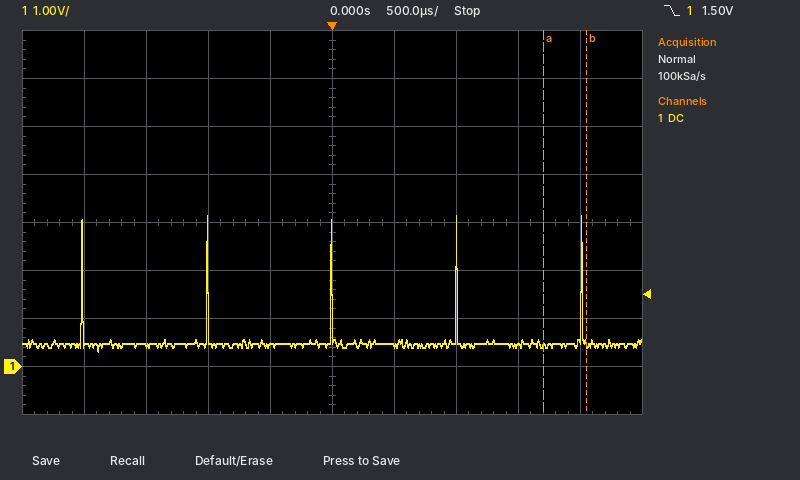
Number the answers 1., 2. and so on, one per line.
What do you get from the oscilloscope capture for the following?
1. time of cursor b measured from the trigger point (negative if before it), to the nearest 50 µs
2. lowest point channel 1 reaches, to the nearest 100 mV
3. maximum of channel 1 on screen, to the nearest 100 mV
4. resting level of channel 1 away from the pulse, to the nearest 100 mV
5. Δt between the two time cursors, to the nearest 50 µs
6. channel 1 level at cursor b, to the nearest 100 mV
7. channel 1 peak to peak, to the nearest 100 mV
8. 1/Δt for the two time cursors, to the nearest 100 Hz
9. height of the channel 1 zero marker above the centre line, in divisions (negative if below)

1. +2.05 ms
2. 300 mV
3. 3.1 V
4. 500 mV
5. 350 µs
6. 500 mV
7. 2.8 V
8. 2.9 kHz
9. -3.0 div
